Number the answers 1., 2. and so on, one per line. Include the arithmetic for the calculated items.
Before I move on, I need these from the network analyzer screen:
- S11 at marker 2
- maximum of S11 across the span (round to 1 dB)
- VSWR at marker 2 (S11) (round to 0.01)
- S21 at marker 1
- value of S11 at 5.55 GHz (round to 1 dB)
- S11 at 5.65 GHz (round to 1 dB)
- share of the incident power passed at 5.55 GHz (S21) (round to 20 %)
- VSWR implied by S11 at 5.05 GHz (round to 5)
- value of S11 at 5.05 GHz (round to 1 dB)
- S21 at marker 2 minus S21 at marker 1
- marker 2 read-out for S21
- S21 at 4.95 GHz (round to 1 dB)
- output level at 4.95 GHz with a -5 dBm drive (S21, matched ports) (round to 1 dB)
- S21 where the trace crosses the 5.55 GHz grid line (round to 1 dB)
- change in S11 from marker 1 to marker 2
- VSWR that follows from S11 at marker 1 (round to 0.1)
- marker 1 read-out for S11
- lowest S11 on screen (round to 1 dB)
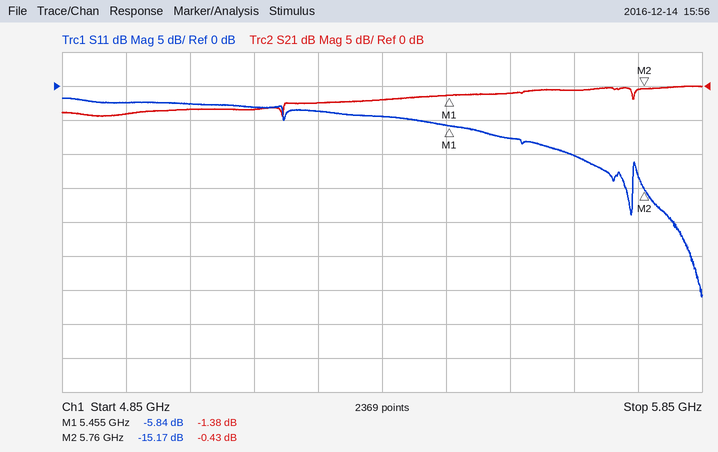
1. -15.17 dB
2. -2 dB
3. (1 + 0.1744)/(1 − 0.1744) ≈ 1.42
4. -1.38 dB
5. -8 dB
6. -10 dB
7. 10^(-1/10) ≈ 79.4 %, so 80 % to the nearest 20 %
8. |Γ| = 10^(-3/20) = 0.7079; VSWR = (1 + 0.7079)/(1 − 0.7079) ≈ 5.85, so 5 to the nearest 5
9. -3 dB
10. -0.43 − (-1.38) = 0.95 dB
11. -0.43 dB
12. -4 dB
13. -5 dBm + (-4 dB) = -9 dBm
14. -1 dB
15. -15.17 − (-5.84) = -9.33 dB
16. (1 + 0.5105)/(1 − 0.5105) ≈ 3.1
17. -5.84 dB
18. -31 dB
